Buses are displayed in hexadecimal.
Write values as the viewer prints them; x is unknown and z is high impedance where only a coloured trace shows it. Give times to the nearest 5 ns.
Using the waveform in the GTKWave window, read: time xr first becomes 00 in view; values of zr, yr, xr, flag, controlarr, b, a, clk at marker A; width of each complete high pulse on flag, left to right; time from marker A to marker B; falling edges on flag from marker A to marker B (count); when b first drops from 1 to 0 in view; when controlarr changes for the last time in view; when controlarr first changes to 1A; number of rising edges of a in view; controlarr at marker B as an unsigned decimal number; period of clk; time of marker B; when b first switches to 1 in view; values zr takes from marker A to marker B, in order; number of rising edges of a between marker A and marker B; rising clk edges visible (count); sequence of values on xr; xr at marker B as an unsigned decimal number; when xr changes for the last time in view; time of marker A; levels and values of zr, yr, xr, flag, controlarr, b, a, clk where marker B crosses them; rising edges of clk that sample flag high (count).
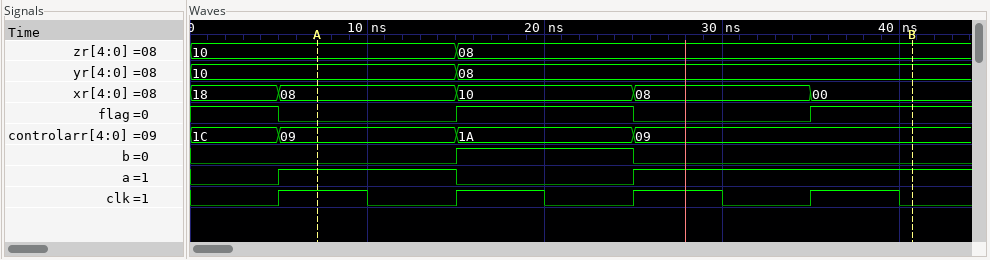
35 ns
zr=10, yr=10, xr=08, flag=0, controlarr=09, b=0, a=1, clk=1
10 ns
35 ns
1
25 ns
25 ns
15 ns
2
9
10 ns
40 ns
15 ns
10, 08
1
4
18, 08, 10, 08, 00
0
35 ns
5 ns
zr=08, yr=08, xr=00, flag=1, controlarr=09, b=0, a=1, clk=0
2
